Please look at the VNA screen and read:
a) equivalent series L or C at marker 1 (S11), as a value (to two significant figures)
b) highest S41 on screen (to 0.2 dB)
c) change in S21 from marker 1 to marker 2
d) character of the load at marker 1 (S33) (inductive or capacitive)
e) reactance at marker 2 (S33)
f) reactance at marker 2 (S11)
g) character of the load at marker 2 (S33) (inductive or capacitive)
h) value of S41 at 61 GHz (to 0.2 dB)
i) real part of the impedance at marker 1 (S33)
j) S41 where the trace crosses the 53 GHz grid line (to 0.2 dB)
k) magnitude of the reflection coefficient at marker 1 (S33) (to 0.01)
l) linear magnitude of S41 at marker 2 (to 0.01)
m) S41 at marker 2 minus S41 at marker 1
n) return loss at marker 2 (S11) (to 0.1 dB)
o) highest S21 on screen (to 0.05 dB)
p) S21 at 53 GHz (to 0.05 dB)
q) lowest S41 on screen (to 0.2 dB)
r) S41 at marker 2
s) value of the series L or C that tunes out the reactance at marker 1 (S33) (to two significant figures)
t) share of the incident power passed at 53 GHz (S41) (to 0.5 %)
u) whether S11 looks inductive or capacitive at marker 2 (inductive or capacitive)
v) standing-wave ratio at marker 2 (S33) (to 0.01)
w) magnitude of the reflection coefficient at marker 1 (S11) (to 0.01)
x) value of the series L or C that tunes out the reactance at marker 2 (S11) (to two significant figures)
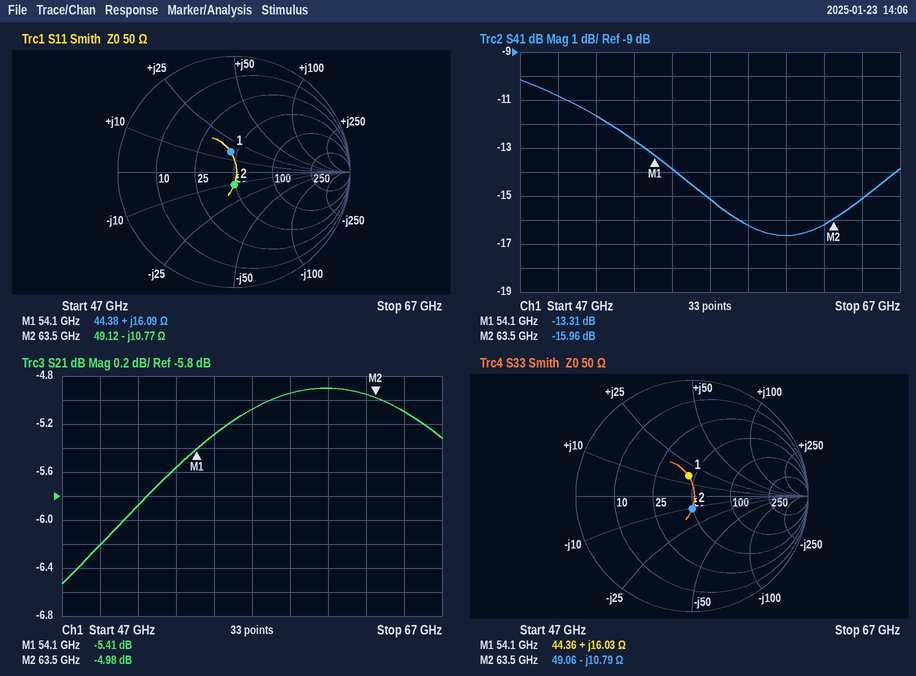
47 pH
-10.2 dB
0.43 dB
inductive
-10.79 Ω
-10.77 Ω
capacitive
-16.6 dB
44.36 Ω
-12.6 dB
0.18
0.16
-2.65 dB
19.3 dB
-4.90 dB
-5.55 dB
-16.6 dB
-15.96 dB
180 fF
5.5 %
capacitive
1.24
0.18
27 pH
